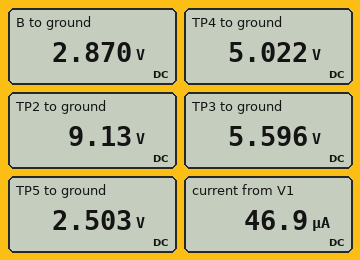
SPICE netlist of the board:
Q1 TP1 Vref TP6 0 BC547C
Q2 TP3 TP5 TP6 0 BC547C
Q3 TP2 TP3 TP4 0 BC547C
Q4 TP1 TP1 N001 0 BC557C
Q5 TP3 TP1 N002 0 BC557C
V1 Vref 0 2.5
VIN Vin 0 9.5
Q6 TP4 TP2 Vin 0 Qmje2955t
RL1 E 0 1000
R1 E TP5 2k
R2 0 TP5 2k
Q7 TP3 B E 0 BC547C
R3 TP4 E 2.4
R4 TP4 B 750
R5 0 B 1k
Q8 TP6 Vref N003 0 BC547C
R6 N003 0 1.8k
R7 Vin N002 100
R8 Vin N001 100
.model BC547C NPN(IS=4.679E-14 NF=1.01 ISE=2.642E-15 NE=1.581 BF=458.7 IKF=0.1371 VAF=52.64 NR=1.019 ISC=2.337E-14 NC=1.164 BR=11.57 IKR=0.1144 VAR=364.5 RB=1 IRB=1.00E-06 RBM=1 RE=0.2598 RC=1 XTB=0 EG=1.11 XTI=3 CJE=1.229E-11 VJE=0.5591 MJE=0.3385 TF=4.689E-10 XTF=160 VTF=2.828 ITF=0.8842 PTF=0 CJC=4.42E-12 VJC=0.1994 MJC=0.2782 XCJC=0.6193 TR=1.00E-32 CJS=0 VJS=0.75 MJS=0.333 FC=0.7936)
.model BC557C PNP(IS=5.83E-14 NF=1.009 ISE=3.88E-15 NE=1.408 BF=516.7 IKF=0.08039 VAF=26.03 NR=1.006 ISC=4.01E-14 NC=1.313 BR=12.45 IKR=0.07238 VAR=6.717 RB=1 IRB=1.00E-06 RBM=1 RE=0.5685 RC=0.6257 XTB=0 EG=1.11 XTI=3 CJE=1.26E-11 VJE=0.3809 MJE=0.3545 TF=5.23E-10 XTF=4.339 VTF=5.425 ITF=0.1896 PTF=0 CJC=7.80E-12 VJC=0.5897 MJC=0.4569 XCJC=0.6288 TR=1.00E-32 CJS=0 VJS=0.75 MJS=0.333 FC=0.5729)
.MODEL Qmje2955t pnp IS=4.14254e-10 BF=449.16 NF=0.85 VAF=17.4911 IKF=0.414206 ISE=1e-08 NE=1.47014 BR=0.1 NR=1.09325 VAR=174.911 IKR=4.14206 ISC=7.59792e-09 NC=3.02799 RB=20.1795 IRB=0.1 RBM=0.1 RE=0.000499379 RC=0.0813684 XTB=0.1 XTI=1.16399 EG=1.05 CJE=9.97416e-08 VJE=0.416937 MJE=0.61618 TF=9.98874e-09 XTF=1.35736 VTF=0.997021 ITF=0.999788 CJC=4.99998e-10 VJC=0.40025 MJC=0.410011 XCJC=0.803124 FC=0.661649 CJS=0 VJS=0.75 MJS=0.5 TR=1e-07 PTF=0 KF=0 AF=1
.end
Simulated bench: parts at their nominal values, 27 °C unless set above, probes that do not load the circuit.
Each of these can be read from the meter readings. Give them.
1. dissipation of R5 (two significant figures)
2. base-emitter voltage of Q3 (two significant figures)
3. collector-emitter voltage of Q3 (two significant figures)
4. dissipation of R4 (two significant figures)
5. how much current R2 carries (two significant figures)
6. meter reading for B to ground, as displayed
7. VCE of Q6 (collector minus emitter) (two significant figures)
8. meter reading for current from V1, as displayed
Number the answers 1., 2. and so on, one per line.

1. 8.2 mW
2. 570 mV
3. 4.1 V
4. 6.2 mW
5. 1.3 mA
6. 2.870 V
7. -4.5 V
8. 46.9 µA
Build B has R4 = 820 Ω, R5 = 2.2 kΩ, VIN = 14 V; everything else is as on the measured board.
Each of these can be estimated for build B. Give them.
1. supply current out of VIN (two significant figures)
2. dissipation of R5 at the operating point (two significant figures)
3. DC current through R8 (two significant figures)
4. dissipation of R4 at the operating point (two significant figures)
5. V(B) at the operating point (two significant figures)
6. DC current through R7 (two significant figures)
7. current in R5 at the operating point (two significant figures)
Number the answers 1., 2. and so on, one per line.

1. 8.9 mA
2. 6.1 mW
3. 470 µA
4. 2.3 mW
5. 3.7 V
6. 520 µA
7. 1.7 mA
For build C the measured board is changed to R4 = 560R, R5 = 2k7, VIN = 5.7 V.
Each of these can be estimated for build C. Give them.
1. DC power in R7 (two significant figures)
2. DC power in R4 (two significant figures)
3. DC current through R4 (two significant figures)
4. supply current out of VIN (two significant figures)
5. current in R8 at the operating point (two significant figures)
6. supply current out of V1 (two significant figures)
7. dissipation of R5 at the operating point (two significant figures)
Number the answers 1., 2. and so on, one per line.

1. 23 µW
2. 1.3 mW
3. 1.5 mA
4. 8.8 mA
5. 500 µA
6. 52 µA
7. 6.4 mW
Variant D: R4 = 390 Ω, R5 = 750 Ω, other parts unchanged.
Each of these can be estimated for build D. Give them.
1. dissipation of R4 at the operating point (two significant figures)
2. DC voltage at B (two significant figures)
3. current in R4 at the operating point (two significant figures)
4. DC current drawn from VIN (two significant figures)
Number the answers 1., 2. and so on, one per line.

1. 7.6 mW
2. 3.3 V
3. 4.4 mA
4. 12 mA
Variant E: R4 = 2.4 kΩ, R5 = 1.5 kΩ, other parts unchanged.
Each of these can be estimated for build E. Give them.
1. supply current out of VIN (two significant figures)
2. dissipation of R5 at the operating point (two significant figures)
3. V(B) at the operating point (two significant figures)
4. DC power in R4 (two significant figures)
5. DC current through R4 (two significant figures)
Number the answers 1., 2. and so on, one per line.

1. 8.5 mA
2. 2.5 mW
3. 1.9 V
4. 4.0 mW
5. 1.3 mA
